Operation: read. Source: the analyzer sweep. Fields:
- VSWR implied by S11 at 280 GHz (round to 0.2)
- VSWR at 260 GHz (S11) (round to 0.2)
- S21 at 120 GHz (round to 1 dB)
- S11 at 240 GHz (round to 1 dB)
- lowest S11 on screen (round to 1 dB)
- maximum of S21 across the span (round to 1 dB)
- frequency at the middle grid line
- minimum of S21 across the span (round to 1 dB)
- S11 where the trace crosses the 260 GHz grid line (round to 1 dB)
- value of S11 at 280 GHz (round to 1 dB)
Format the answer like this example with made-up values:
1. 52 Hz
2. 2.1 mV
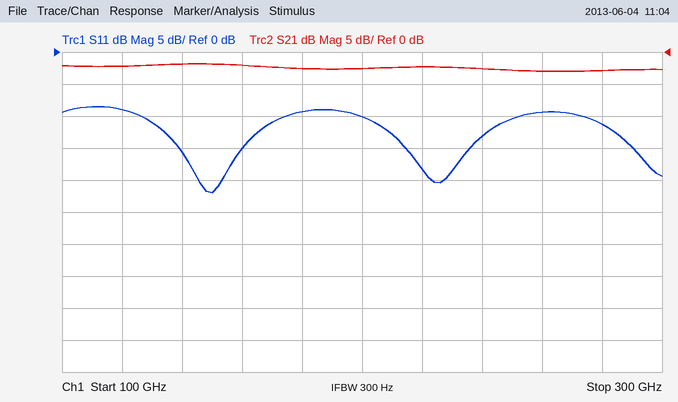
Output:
1. 1.8
2. 2.0
3. -2 dB
4. -13 dB
5. -22 dB
6. -2 dB
7. 200 GHz
8. -3 dB
9. -9 dB
10. -11 dB
